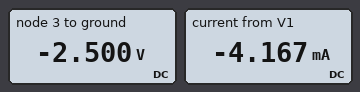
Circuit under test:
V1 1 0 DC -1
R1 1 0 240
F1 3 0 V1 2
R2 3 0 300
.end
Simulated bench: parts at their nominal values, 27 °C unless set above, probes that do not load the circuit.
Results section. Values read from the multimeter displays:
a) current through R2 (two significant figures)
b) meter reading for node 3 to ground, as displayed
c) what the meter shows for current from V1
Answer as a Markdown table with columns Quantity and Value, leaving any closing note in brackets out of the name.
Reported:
| Quantity | Value |
|---|---|
| current through R2 | 8.3 mA |
| meter reading for node 3 to ground, as displayed | -2.500 V |
| what the meter shows for current from V1 | -4.167 mA |
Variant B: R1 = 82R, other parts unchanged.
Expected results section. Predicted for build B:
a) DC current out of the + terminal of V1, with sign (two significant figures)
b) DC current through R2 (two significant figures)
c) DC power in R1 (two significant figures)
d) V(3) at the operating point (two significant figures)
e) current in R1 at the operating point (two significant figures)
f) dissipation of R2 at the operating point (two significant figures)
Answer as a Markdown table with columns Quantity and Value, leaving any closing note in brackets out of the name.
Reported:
| Quantity | Value |
|---|---|
| DC current out of the + terminal of V1, with sign | -12 mA |
| DC current through R2 | 24 mA |
| DC power in R1 | 12 mW |
| V(3) at the operating point | -7.3 V |
| current in R1 at the operating point | 12 mA |
| dissipation of R2 at the operating point | 180 mW |
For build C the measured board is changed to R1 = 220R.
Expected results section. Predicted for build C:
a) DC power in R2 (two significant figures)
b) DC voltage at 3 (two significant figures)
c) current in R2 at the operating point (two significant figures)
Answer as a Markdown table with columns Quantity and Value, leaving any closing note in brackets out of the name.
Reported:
| Quantity | Value |
|---|---|
| DC power in R2 | 25 mW |
| DC voltage at 3 | -2.7 V |
| current in R2 at the operating point | 9.1 mA |
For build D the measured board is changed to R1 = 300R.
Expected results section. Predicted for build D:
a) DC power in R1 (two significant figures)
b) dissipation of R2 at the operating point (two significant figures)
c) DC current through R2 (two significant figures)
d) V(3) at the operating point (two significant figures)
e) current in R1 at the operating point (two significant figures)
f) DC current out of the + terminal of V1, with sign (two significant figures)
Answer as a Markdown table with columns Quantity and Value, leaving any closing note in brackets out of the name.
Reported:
| Quantity | Value |
|---|---|
| DC power in R1 | 3.3 mW |
| dissipation of R2 at the operating point | 13 mW |
| DC current through R2 | 6.7 mA |
| V(3) at the operating point | -2.0 V |
| current in R1 at the operating point | 3.3 mA |
| DC current out of the + terminal of V1, with sign | -3.3 mA |
